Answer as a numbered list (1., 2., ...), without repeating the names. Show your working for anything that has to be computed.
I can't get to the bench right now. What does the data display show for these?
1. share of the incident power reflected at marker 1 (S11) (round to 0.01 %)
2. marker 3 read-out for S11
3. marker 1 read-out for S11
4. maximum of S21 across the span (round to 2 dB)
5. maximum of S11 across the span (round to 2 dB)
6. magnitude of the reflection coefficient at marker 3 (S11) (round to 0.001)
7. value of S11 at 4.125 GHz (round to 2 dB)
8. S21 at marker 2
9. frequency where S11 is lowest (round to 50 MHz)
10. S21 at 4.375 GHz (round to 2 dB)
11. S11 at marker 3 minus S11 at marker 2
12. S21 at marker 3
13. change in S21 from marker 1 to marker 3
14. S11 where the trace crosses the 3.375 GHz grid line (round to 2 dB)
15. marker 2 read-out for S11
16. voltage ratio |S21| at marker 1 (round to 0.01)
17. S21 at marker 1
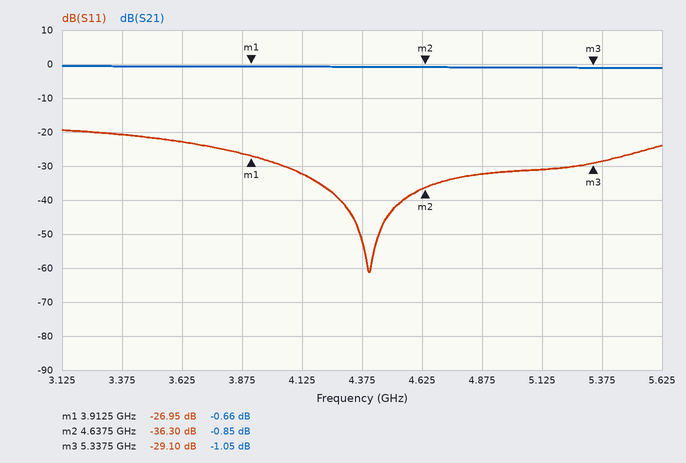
1. 10^(-26.95/10) ≈ 0.20 %
2. -29.10 dB
3. -26.95 dB
4. 0 dB
5. -20 dB
6. 10^(-29.1/20) ≈ 0.035
7. -32 dB
8. -0.85 dB
9. 4.40 GHz
10. 0 dB
11. -29.1 − (-36.3) = 7.20 dB
12. -1.05 dB
13. -1.05 − (-0.66) = -0.39 dB
14. -20 dB
15. -36.30 dB
16. 10^(-0.66/20) ≈ 0.93
17. -0.66 dB
